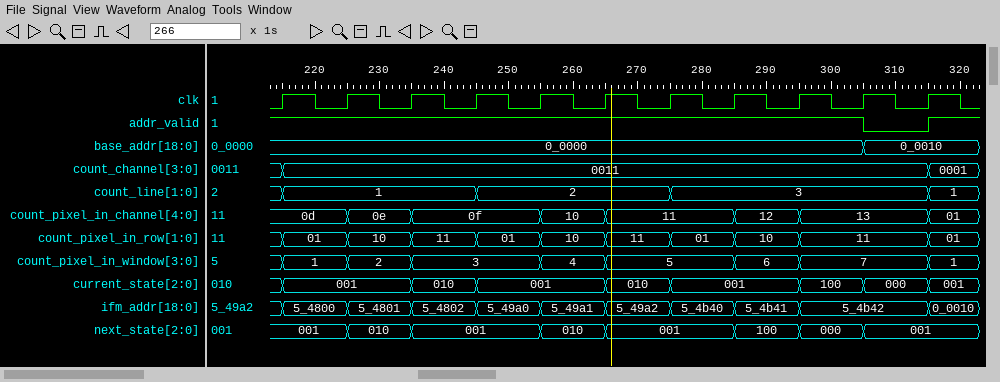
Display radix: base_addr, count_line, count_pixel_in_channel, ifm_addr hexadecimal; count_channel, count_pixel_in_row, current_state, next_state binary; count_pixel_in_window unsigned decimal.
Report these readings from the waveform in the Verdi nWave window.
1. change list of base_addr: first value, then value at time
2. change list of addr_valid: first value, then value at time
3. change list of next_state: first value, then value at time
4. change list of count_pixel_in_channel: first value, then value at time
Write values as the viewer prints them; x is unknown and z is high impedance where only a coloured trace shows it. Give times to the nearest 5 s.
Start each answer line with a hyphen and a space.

- 0_0000, 0_0010 at 305 s
- 1, 0 at 305 s, 1 at 315 s
- 001, 010 at 225 s, 001 at 235 s, 010 at 255 s, 001 at 265 s, 100 at 285 s, 000 at 295 s, 001 at 305 s
- 0d, 0e at 225 s, 0f at 235 s, 10 at 255 s, 11 at 265 s, 12 at 285 s, 13 at 295 s, 01 at 315 s
